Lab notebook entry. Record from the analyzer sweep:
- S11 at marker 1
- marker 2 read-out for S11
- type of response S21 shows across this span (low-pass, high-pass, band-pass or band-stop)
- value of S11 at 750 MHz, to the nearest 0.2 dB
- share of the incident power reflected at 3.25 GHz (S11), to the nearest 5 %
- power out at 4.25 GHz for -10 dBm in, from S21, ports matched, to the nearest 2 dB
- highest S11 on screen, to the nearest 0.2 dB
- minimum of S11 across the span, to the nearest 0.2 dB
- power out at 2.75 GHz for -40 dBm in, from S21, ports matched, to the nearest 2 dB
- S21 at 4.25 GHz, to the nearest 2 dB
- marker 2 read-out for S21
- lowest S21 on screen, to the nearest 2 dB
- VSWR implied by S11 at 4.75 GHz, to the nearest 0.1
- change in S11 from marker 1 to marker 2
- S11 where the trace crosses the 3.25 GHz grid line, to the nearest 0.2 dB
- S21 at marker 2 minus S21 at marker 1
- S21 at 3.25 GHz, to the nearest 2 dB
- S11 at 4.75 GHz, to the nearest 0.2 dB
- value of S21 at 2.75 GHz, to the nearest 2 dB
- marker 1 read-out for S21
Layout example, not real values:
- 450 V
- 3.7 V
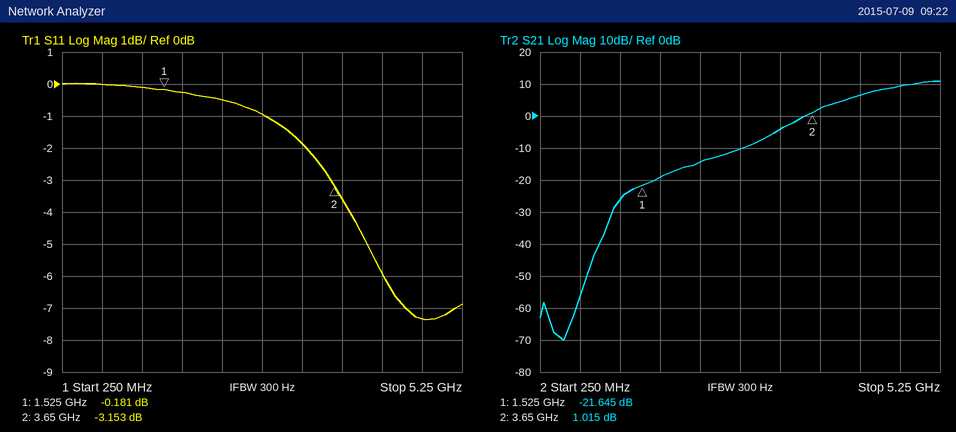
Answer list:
- -0.181 dB
- -3.153 dB
- high-pass
- 0.0 dB
- 65 %
- -4 dBm
- 0.0 dB
- -7.4 dB
- -50 dBm
- 6 dB
- 1.015 dB
- -70 dB
- 2.5
- -2.972 dB
- -1.8 dB
- 22.660 dB
- -4 dB
- -7.4 dB
- -10 dB
- -21.645 dB
